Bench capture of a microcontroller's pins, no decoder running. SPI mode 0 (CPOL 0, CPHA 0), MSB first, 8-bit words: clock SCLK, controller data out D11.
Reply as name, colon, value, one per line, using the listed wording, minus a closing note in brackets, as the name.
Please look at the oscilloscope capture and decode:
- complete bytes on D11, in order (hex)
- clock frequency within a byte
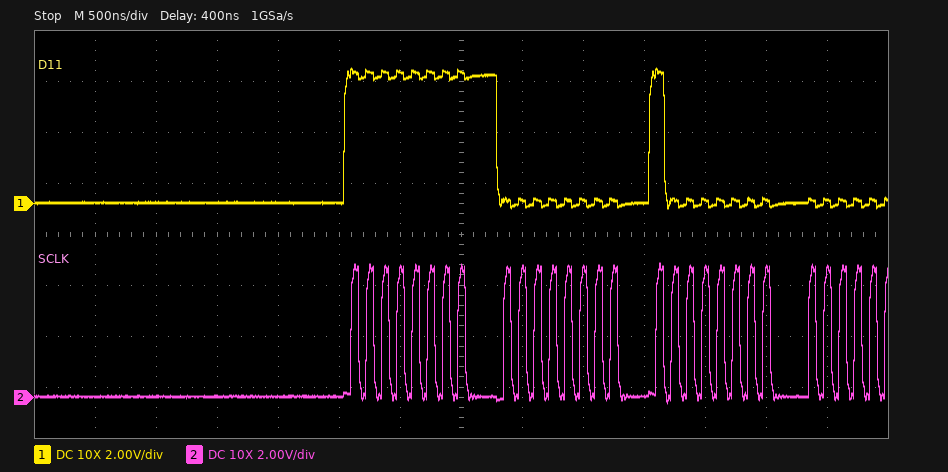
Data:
complete bytes on D11, in order: 0xFF 0x00 0x80
clock frequency within a byte: 8 MHz
